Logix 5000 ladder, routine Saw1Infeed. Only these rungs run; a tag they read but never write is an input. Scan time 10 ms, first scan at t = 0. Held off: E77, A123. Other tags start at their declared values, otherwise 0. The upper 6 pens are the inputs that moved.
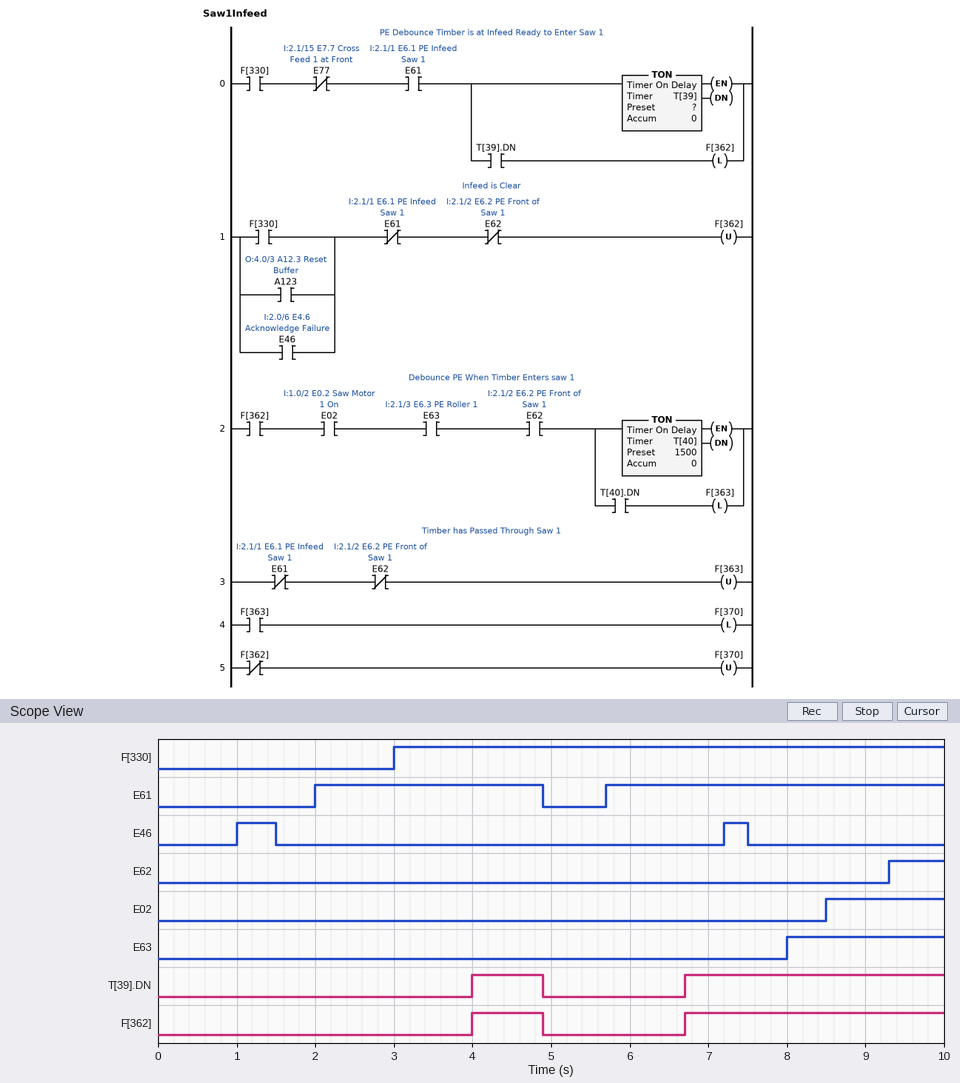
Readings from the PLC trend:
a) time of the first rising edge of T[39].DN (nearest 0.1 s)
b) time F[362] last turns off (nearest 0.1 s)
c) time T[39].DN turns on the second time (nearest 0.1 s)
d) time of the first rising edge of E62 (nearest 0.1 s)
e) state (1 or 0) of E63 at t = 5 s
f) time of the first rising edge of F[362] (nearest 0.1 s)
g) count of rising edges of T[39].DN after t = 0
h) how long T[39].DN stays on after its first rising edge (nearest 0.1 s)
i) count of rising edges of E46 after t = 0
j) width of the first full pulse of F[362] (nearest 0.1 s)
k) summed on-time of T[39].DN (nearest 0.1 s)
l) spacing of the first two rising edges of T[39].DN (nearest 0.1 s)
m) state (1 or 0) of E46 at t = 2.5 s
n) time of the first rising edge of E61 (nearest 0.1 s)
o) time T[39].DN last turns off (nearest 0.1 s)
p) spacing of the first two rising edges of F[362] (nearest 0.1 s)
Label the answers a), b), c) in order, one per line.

a) 4.0 s
b) 4.9 s
c) 6.7 s
d) 9.3 s
e) 0
f) 4.0 s
g) 2
h) 0.9 s
i) 2
j) 0.9 s
k) 4.2 s
l) 2.7 s
m) 0
n) 2.0 s
o) 4.9 s
p) 2.7 s
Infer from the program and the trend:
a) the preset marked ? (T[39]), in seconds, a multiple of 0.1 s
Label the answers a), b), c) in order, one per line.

a) 1.0 s
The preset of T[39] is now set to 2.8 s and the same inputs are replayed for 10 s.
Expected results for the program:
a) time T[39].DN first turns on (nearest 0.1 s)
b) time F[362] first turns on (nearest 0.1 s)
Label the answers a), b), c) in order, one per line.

a) 8.5 s
b) 8.5 s
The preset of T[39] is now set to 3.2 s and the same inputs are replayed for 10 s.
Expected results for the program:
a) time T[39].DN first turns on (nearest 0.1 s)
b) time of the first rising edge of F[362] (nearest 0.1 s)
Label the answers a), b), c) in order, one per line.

a) 8.9 s
b) 8.9 s
